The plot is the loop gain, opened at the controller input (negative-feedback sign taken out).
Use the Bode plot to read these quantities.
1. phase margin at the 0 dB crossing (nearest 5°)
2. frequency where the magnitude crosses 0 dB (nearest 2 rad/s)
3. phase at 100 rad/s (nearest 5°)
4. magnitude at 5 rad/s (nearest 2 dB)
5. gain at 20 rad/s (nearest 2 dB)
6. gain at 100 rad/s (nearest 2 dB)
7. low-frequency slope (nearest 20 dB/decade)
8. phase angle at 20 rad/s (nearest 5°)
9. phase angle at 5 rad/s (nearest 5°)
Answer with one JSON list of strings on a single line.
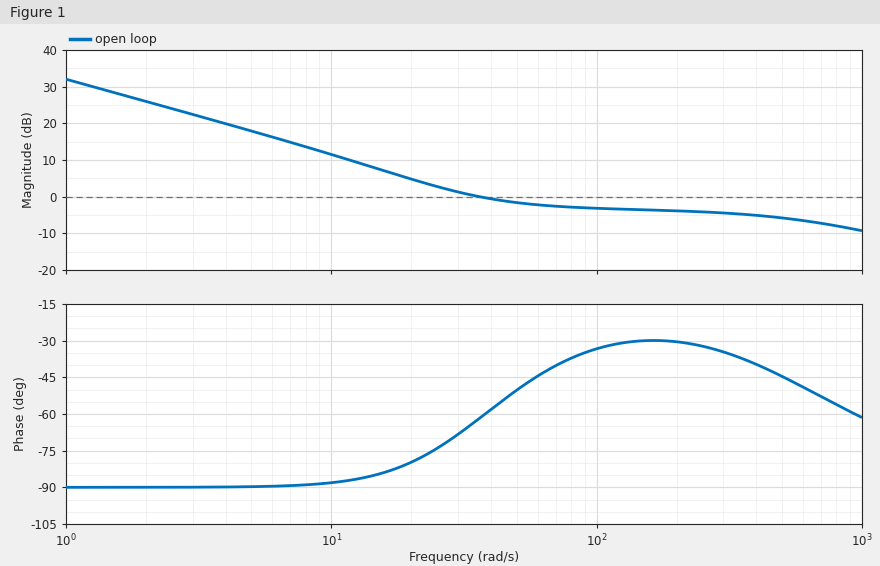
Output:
["120°", "36 rad/s", "-35°", "18 dB", "4 dB", "-4 dB", "-20 dB/decade", "-80°", "-90°"]
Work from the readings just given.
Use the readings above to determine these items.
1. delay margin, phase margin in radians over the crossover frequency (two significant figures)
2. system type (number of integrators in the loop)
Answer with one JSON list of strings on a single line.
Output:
["0.058 s", "1"]
